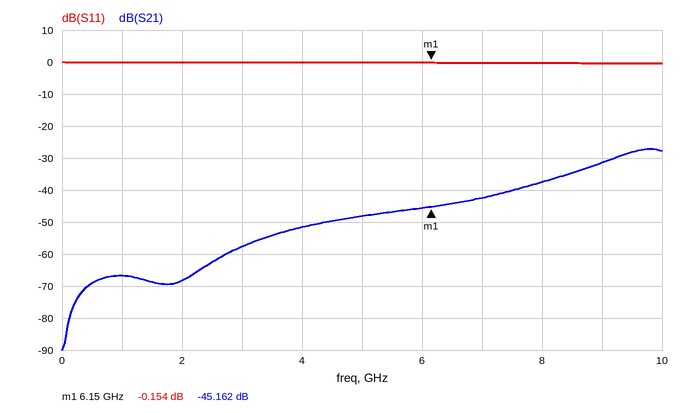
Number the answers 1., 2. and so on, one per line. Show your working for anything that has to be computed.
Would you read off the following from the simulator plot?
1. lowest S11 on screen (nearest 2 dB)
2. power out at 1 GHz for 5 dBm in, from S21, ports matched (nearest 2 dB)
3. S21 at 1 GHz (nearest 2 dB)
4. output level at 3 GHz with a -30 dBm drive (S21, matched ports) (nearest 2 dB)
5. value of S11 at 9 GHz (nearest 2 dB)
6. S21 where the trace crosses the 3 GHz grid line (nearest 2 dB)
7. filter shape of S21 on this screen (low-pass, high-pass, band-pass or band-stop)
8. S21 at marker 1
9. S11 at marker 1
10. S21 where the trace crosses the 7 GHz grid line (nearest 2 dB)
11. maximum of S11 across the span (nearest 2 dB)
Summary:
1. 0 dB
2. 5 dBm + (-66 dB) = -62 dBm
3. -66 dB
4. -30 dBm + (-58 dB) = -88 dBm
5. 0 dB
6. -58 dB
7. high-pass
8. -45.162 dB
9. -0.154 dB
10. -42 dB
11. 0 dB
